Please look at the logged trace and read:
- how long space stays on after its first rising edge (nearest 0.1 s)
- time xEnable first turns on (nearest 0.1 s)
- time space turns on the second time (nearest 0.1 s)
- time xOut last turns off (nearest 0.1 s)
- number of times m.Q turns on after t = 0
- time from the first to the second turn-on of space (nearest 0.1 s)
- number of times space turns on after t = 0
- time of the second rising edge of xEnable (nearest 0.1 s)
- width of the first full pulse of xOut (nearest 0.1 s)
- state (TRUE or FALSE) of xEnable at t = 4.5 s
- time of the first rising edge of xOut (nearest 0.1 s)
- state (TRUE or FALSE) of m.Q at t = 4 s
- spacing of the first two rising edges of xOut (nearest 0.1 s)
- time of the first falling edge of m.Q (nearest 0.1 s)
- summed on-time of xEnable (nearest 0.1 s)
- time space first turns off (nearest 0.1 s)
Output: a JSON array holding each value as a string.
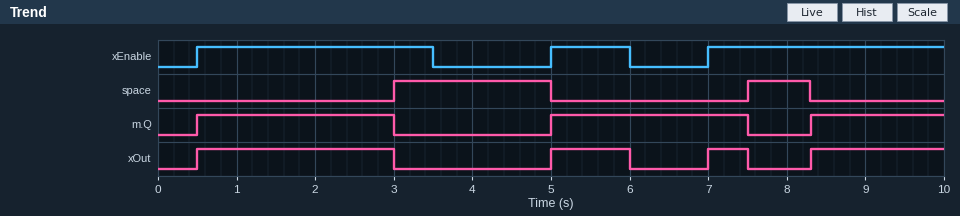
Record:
["2.0 s", "0.5 s", "7.5 s", "7.5 s", "3", "4.5 s", "2", "5.0 s", "2.5 s", "FALSE", "0.5 s", "FALSE", "4.5 s", "3.0 s", "7.0 s", "5.0 s"]
